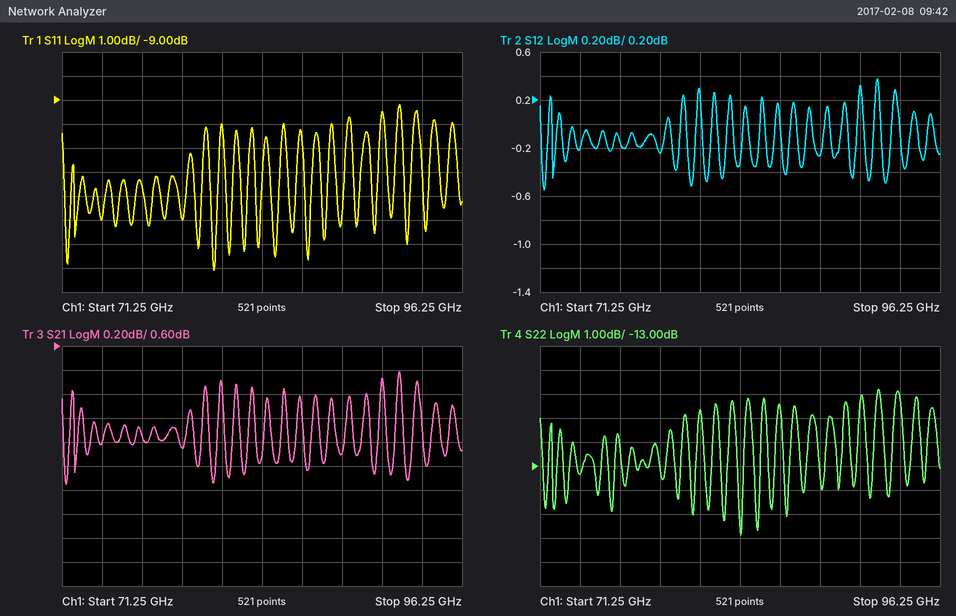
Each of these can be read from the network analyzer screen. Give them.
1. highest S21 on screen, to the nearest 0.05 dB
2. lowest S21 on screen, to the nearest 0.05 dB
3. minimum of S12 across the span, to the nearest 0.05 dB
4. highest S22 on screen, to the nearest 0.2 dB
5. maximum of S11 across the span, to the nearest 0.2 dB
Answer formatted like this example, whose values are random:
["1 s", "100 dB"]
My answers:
["0.40 dB", "-0.55 dB", "-0.55 dB", "-9.8 dB", "-9.2 dB"]
